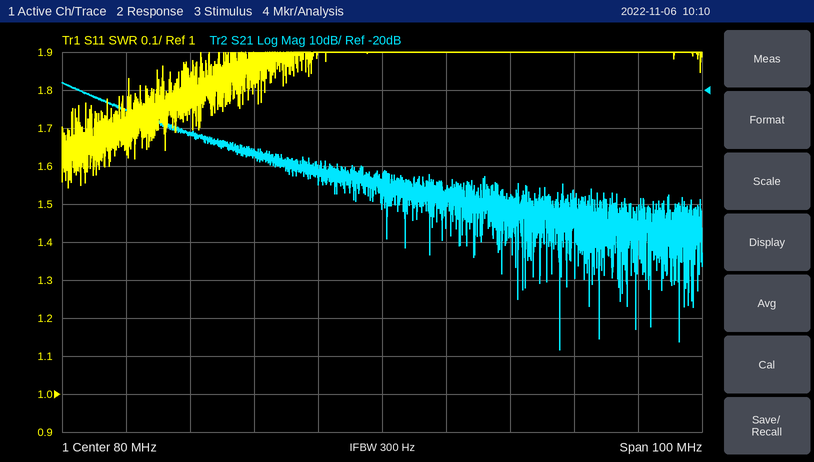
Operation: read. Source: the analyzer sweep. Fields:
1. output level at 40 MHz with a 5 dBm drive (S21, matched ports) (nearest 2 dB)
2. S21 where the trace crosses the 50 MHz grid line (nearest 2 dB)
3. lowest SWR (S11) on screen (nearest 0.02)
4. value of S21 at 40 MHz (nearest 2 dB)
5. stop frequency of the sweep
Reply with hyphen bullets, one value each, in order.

- -20 dBm
- -32 dB
- 1.54
- -26 dB
- 130 MHz
